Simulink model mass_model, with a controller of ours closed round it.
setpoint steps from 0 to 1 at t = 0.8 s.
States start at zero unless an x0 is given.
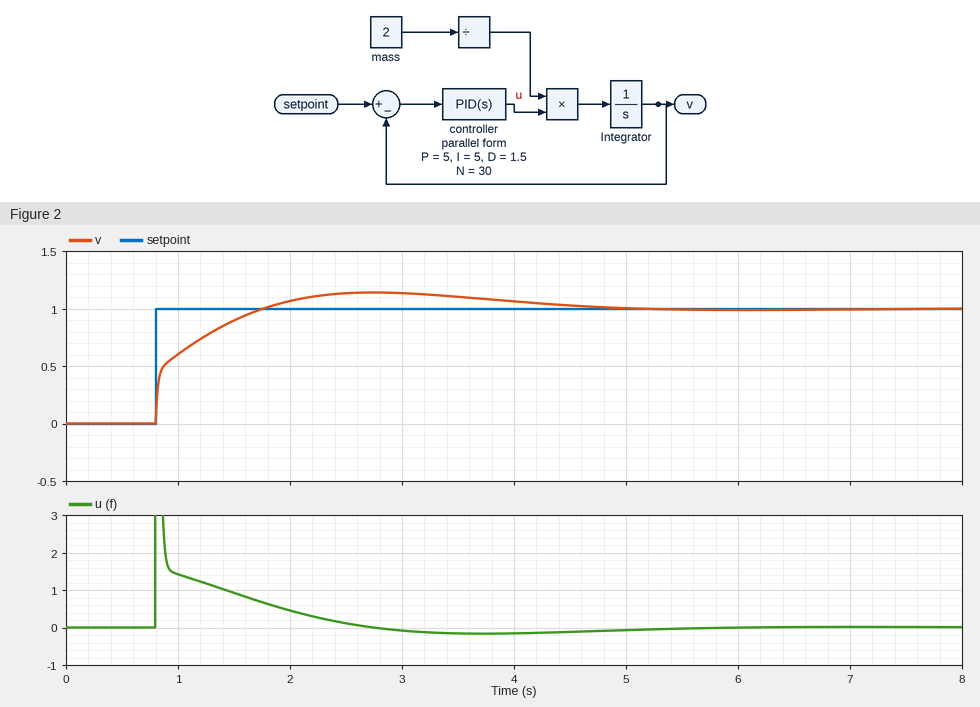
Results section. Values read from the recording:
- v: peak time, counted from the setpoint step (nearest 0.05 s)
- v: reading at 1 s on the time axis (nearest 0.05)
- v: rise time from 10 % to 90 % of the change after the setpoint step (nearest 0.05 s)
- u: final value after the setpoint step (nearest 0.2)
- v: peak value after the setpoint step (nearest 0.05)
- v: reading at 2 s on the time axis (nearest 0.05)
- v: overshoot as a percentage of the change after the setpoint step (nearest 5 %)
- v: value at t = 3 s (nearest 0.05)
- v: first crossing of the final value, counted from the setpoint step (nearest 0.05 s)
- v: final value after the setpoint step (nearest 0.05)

1.95 s
0.60
0.70 s
0.0
1.15
1.05
15 %
1.15
0.95 s
1.00
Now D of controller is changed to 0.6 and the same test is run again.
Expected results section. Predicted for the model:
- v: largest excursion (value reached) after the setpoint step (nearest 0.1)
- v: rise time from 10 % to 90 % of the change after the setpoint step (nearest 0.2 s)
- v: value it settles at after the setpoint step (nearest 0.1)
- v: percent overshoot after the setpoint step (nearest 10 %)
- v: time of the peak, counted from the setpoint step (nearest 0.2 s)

1.2
0.6 s
1.0
20 %
1.6 s
